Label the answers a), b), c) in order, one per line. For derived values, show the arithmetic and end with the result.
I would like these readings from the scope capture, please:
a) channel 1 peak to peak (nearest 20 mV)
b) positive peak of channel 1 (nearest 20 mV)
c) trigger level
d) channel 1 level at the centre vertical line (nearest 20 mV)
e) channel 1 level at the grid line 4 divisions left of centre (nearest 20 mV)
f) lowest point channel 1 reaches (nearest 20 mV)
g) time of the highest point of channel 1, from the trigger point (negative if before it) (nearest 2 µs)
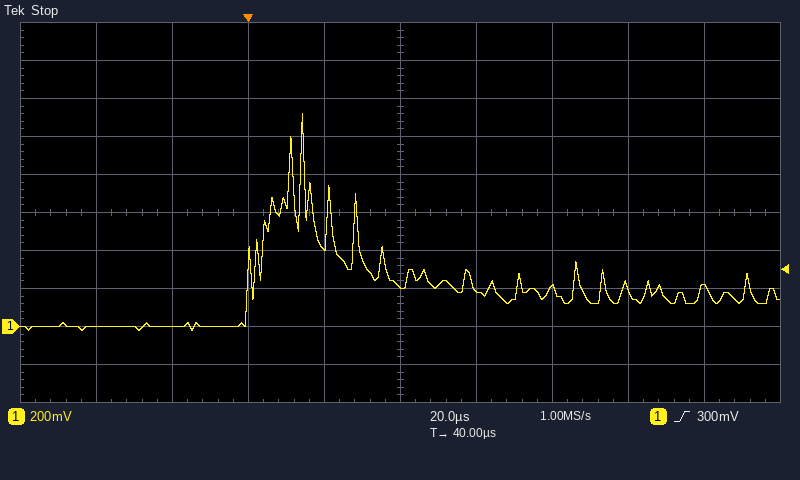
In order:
a) 1.12 V − (-20 mV) = 1.14 V
b) 1.12 V
c) 300 mV
d) 220 mV
e) 0 mV
f) -20 mV
g) +14 µs
